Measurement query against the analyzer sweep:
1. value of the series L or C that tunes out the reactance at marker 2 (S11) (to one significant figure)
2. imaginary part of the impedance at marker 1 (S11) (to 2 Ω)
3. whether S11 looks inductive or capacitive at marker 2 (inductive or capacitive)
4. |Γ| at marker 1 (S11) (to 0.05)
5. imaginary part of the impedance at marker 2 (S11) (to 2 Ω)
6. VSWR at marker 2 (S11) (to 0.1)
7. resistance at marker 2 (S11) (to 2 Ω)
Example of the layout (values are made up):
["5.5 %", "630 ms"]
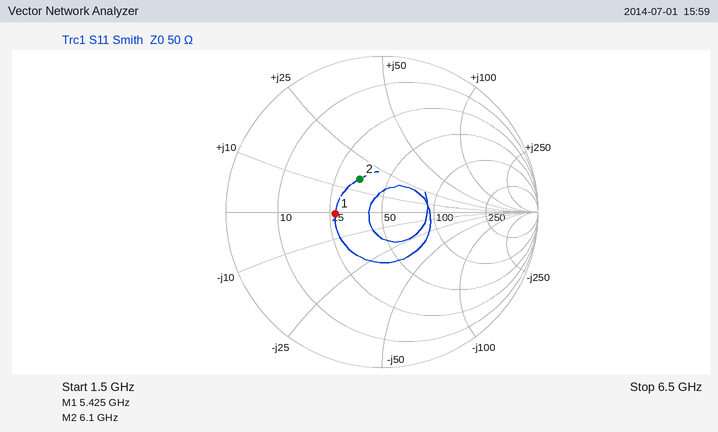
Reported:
["2 pF", "0 Ω", "inductive", "0.30", "+16 Ω", "1.7", "34 Ω"]
